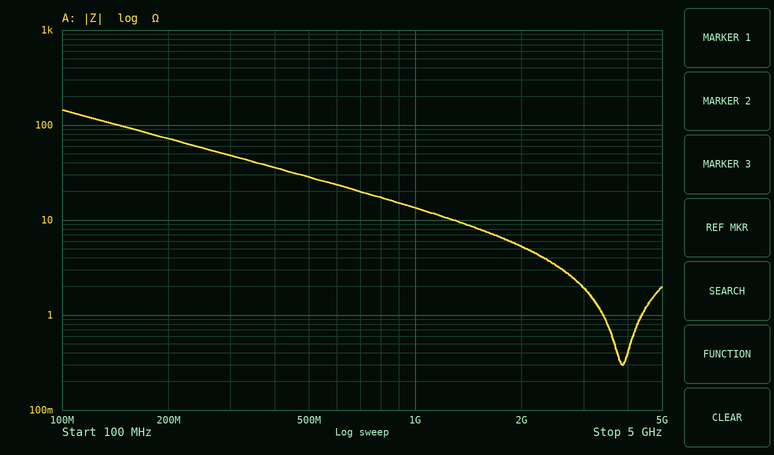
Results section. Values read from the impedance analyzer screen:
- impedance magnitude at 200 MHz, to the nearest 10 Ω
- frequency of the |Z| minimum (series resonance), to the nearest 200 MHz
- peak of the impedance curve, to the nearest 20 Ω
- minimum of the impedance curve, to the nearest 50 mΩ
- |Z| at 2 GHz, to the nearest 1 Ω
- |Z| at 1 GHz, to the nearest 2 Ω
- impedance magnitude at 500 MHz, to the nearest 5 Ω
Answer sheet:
70 Ω
3.8 GHz
140 Ω
300 mΩ
5 Ω
14 Ω
30 Ω
